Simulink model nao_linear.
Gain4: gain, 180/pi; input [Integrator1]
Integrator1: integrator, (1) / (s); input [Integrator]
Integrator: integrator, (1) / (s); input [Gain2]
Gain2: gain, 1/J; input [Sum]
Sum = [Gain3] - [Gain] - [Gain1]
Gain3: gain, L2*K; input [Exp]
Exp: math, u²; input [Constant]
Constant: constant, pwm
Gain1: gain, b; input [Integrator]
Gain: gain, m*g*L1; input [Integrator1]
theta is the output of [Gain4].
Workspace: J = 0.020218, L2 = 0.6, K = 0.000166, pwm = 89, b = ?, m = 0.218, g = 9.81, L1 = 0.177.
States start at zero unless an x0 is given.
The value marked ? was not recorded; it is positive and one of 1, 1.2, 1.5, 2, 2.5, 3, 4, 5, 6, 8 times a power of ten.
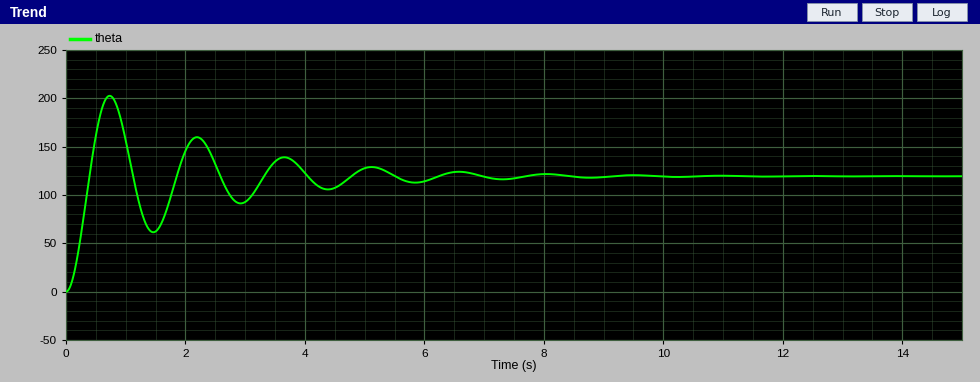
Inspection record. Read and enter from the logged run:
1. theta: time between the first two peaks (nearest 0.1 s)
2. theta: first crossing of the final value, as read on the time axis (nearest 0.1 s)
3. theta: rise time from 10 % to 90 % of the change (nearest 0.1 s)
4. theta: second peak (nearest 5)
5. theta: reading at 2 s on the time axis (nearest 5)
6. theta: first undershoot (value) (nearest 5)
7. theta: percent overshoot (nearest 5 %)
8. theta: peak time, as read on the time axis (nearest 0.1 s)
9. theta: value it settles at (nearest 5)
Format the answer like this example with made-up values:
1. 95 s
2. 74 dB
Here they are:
1. 1.5 s
2. 0.4 s
3. 0.3 s
4. 160
5. 145
6. 60
7. 70 %
8. 0.7 s
9. 120
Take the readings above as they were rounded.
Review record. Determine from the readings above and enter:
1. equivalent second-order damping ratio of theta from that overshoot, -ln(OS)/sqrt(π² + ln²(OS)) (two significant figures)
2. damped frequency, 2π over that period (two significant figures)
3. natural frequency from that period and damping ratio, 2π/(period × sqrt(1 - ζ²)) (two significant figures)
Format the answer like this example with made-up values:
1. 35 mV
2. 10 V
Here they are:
1. 0.11
2. 4.2 rad/s
3. 4.2 rad/s
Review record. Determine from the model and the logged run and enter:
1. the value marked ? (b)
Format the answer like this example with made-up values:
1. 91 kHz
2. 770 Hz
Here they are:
1. 0.02
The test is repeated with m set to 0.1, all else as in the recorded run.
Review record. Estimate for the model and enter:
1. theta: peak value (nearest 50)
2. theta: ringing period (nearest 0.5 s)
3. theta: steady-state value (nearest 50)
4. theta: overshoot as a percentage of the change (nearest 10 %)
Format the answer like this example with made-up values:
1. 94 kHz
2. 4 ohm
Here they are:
1. 400
2. 2.0 s
3. 250
4. 60 %
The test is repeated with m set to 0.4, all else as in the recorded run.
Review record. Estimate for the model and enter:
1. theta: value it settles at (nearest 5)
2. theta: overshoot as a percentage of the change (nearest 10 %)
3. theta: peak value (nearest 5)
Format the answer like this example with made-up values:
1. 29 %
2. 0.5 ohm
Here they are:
1. 65
2. 80 %
3. 115
